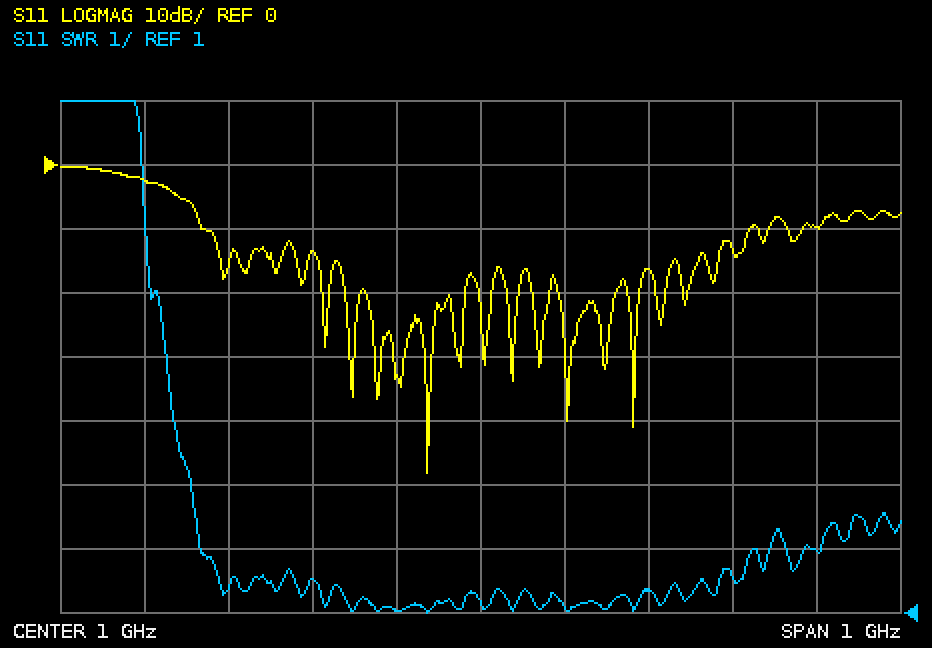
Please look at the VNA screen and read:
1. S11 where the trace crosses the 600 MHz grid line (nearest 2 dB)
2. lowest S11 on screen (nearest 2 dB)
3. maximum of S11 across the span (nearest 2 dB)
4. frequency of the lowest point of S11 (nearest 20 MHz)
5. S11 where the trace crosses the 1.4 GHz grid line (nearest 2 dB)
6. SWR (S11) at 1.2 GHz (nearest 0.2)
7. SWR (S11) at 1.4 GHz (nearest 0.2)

-2 dB
-48 dB
0 dB
940 MHz
-10 dB
1.4
2.0
